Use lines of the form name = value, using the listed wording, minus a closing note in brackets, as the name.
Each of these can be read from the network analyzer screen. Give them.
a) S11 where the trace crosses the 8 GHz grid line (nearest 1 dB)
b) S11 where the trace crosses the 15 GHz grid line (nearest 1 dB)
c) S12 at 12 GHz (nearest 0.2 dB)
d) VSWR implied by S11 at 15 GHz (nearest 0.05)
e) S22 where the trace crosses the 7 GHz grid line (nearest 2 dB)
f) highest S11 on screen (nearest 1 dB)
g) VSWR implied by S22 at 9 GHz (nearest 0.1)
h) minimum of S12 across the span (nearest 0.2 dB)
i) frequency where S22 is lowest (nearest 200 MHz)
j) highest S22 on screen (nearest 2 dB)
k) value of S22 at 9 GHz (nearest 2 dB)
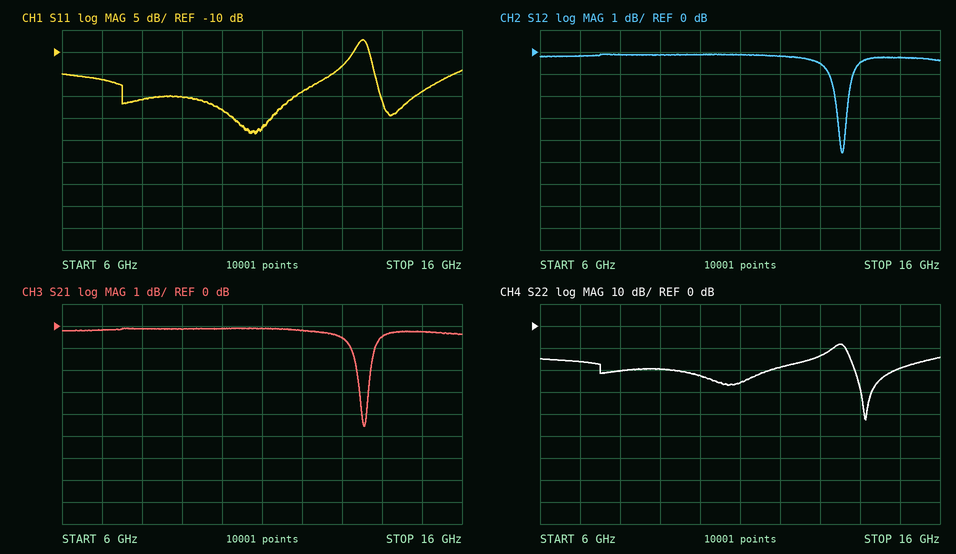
S11 where the trace crosses the 8 GHz grid line = -21 dB
S11 where the trace crosses the 15 GHz grid line = -19 dB
S12 at 12 GHz = -0.2 dB
VSWR implied by S11 at 15 GHz = 1.25
S22 where the trace crosses the 7 GHz grid line = -16 dB
highest S11 on screen = -7 dB
VSWR implied by S22 at 9 GHz = 1.2
minimum of S12 across the span = -4.6 dB
frequency where S22 is lowest = 14.2 GHz
highest S22 on screen = -8 dB
value of S22 at 9 GHz = -20 dB
